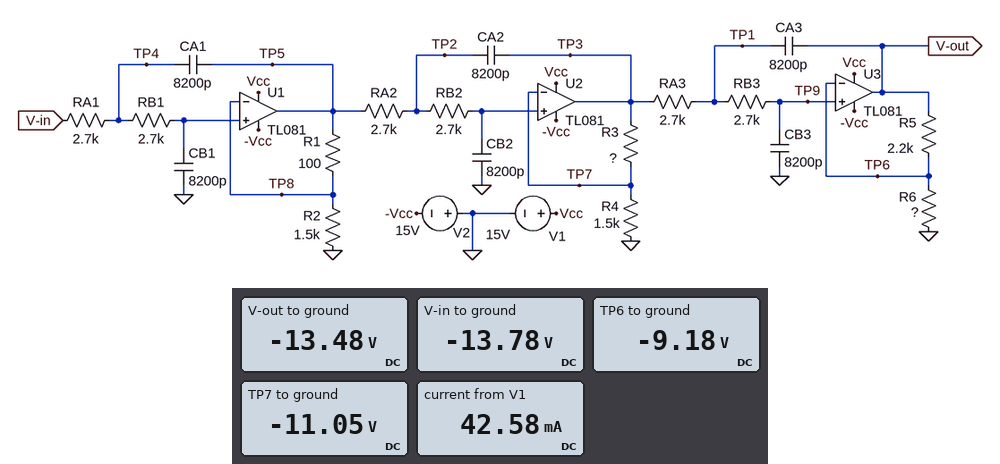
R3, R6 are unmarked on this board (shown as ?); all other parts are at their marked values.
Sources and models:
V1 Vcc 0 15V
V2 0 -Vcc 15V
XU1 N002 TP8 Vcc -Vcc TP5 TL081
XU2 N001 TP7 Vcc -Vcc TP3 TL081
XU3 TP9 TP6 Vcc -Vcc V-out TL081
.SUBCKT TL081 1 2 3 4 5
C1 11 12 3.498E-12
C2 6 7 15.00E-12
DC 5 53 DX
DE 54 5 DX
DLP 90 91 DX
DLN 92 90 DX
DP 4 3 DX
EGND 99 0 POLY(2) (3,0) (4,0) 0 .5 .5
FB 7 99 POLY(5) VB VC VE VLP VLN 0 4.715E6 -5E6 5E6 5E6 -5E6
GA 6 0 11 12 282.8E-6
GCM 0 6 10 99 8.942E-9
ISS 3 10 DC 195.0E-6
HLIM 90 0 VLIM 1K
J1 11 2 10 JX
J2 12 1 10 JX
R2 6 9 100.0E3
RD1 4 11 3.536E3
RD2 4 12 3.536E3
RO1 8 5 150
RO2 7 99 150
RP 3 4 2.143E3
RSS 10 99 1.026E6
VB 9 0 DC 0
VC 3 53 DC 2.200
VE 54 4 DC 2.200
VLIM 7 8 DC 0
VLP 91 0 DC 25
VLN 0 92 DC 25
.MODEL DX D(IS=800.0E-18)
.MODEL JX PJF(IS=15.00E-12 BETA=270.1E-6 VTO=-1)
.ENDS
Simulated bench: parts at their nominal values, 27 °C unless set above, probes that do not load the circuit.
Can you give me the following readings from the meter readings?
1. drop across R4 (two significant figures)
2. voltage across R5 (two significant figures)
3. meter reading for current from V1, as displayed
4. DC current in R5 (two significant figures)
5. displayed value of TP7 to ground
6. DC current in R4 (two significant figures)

11 V
4.3 V
42.58 mA
2.0 mA
-11.05 V
7.4 mA
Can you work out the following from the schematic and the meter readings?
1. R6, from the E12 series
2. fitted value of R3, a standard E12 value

4.7 kΩ
330 Ω
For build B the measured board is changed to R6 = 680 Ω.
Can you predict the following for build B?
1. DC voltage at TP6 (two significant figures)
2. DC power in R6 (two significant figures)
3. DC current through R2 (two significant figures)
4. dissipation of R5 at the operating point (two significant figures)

-3.2 V
15 mW
8.4 mA
48 mW
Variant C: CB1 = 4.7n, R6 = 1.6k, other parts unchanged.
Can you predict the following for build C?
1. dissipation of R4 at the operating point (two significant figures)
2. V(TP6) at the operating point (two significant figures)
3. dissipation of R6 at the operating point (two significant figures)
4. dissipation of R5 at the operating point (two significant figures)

81 mW
-5.7 V
20 mW
28 mW
